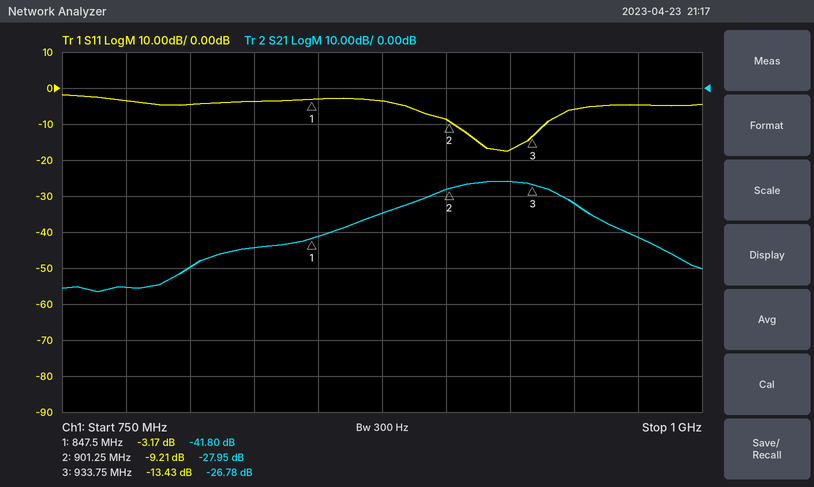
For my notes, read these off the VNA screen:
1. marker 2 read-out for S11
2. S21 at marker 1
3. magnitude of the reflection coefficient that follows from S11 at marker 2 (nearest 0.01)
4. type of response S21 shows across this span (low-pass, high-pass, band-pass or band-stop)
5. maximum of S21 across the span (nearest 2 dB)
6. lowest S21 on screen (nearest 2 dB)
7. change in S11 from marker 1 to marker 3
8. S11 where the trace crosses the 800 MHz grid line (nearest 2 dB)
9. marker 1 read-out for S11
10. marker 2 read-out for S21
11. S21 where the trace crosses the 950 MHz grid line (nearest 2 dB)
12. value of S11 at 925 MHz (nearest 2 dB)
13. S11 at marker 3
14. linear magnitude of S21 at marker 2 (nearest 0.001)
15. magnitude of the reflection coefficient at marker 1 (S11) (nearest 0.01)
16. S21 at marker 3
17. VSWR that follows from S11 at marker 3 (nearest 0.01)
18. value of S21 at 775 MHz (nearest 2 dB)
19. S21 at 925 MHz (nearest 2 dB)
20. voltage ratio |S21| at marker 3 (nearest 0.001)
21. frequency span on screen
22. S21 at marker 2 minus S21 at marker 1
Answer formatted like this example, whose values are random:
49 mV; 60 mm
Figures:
-9.21 dB; -41.80 dB; 0.35; band-pass; -26 dB; -56 dB; -10.26 dB; -4 dB; -3.17 dB; -27.95 dB; -32 dB; -18 dB; -13.43 dB; 0.040; 0.69; -26.78 dB; 1.54; -56 dB; -26 dB; 0.046; 250 MHz; 13.85 dB
